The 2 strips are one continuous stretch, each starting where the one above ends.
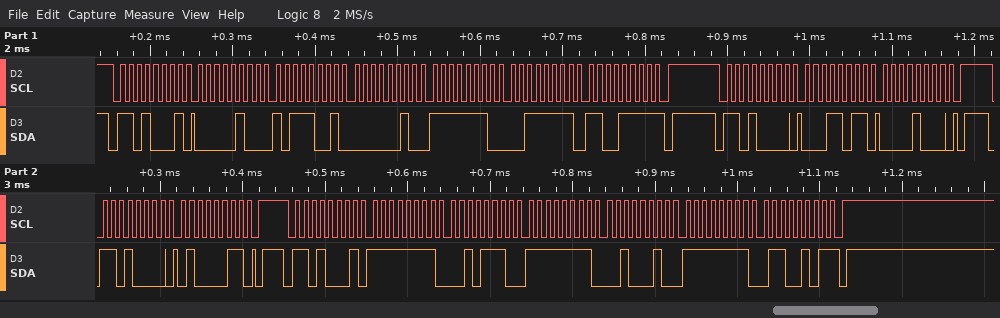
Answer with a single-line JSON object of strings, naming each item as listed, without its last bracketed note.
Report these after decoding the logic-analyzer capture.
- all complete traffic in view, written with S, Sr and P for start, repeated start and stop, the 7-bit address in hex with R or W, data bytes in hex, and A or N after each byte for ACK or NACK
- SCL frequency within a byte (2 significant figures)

{"all complete traffic in view, written with S, Sr and P for start, repeated start and stop, the 7-bit address in hex with R or W, data bytes in hex, and A or N after each byte for ACK or NACK": "S 68R A 04 A B9 A 02 A FE A 3F A CF N P S 68W A 1B A 08 A P S 68W A 43 A P S 68R A FF A 2E A FF A 22 A FF A 65 N P", "SCL frequency within a byte": "100 kHz"}
